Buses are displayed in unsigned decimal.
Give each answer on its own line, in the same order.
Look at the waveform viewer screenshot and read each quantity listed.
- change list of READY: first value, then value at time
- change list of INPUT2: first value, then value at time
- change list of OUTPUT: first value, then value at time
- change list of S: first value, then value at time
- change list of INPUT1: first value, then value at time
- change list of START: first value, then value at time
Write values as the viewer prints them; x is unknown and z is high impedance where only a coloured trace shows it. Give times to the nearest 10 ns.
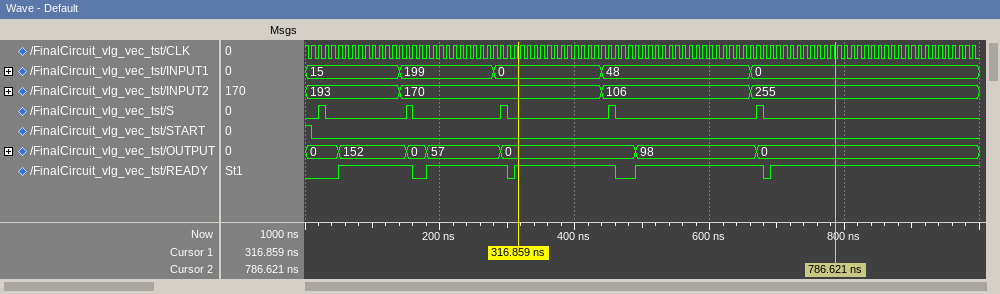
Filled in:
0, 1 at 50 ns, 0 at 160 ns, 1 at 180 ns, 0 at 300 ns, 1 at 310 ns, 0 at 460 ns, 1 at 490 ns, 0 at 680 ns, 1 at 690 ns
193, 170 at 140 ns, 106 at 440 ns, 255 at 660 ns
0, 152 at 50 ns, 0 at 150 ns, 57 at 180 ns, 0 at 290 ns, 98 at 490 ns, 0 at 670 ns
0, 1 at 20 ns, 0 at 30 ns, 1 at 150 ns, 0 at 160 ns, 1 at 290 ns, 0 at 300 ns, 1 at 450 ns, 0 at 460 ns, 1 at 670 ns, 0 at 680 ns
15, 199 at 140 ns, 0 at 280 ns, 48 at 440 ns, 0 at 660 ns
1, 0 at 10 ns
